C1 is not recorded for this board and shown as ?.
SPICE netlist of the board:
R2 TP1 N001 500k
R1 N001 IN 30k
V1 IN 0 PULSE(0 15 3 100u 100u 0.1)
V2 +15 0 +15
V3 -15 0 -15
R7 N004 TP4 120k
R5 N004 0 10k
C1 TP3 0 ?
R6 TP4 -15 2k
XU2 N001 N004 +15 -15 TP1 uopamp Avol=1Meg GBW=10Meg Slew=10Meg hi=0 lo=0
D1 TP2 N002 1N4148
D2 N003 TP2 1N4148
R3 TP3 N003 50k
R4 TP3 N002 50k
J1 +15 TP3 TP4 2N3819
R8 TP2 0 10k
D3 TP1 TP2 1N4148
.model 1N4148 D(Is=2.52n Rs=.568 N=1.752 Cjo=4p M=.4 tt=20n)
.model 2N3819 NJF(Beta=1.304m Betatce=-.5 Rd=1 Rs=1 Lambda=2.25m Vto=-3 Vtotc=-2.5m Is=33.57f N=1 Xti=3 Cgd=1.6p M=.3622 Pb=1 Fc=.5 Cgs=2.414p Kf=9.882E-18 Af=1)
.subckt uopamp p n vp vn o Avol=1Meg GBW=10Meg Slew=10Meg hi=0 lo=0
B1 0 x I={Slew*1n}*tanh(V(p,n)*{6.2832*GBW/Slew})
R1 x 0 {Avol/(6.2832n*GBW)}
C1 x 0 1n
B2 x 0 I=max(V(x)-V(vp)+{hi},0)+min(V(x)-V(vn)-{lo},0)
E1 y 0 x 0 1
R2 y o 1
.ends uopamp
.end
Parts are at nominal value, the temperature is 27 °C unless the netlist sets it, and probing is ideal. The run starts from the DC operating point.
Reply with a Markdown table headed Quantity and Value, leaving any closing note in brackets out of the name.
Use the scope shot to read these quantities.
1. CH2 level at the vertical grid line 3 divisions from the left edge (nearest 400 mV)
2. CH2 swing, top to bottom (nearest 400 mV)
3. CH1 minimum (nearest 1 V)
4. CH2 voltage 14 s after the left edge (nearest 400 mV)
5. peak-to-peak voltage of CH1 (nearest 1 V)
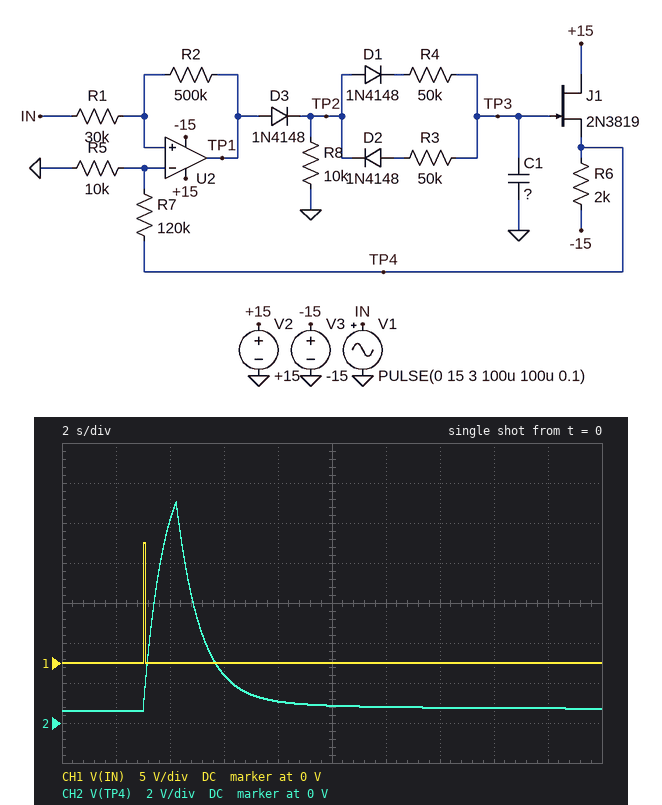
| Quantity | Value |
|---|---|
| CH2 level at the vertical grid line 3 divisions from the left edge | 2.4 V |
| CH2 swing, top to bottom | 10.4 V |
| CH1 minimum | 0 V |
| CH2 voltage 14 s after the left edge | 800 mV |
| peak-to-peak voltage of CH1 | 15 V |
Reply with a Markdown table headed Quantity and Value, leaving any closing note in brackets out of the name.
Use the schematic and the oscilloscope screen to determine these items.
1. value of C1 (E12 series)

| Quantity | Value |
|---|---|
| value of C1 | 15 µF |
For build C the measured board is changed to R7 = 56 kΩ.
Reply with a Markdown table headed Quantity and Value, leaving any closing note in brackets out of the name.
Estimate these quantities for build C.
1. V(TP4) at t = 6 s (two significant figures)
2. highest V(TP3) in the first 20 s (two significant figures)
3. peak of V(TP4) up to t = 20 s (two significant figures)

| Quantity | Value |
|---|---|
| V(TP4) at t = 6 s | 1.2 V |
| highest V(TP3) in the first 20 s | 5.4 V |
| peak of V(TP4) up to t = 20 s | 5.6 V |
